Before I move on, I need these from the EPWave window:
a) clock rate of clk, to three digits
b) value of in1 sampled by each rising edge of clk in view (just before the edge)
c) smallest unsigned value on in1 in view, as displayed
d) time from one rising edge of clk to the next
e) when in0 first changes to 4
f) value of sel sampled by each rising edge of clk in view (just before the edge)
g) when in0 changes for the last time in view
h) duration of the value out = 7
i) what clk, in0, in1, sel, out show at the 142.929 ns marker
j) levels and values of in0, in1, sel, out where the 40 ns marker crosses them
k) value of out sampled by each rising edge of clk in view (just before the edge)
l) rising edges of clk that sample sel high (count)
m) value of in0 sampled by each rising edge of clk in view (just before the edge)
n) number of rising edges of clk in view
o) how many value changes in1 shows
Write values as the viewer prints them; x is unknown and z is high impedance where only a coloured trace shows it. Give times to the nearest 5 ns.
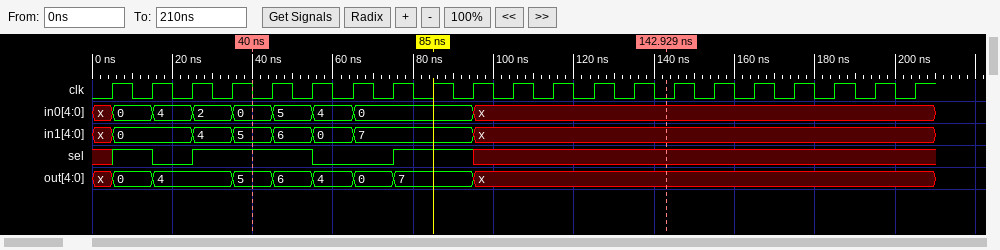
100 MHz
x, 0, 0, 4, 5, 6, 0, 7, 7, 7, x, x, x, x, x, x, x, x, x, x, x
0
10 ns
15 ns
x 1 0 1 1 1 0 0 1 1 x x x x x x x x x x x
95 ns
20 ns
clk=0, in0=x, in1=x, sel=x, out=x
in0=0, in1=5, sel=1, out=5
x, 0, 4, 4, 5, 6, 4, 0, 7, 7, x, x, x, x, x, x, x, x, x, x, x
6
x, 0, 4, 2, 0, 5, 4, 0, 0, 0, x, x, x, x, x, x, x, x, x, x, x
21
7
